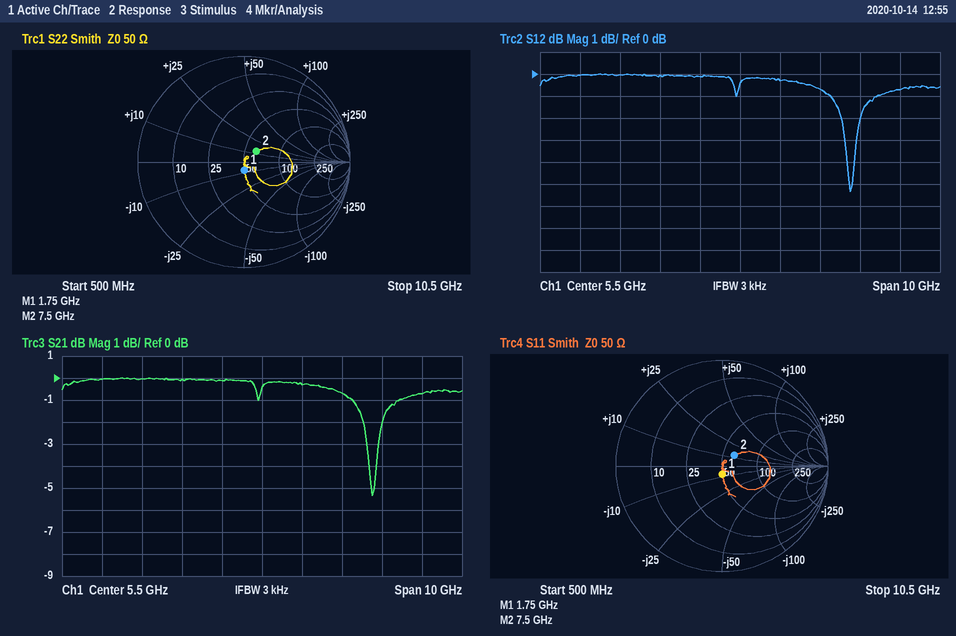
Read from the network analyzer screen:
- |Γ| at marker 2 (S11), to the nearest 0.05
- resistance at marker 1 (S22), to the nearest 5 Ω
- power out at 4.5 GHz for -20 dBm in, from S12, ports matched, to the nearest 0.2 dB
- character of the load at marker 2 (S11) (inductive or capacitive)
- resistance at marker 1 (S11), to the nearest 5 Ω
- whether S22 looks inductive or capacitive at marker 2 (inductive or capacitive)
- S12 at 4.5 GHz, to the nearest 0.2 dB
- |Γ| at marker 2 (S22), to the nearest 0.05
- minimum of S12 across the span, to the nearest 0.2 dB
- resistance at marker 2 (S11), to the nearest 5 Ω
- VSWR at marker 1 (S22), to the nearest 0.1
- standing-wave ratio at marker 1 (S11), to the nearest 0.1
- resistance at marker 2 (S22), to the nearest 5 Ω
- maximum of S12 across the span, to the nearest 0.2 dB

0.15
50 Ω
-20.2 dBm
inductive
50 Ω
inductive
-0.2 dB
0.15
-5.4 dB
60 Ω
1.2
1.2
60 Ω
0.0 dB
